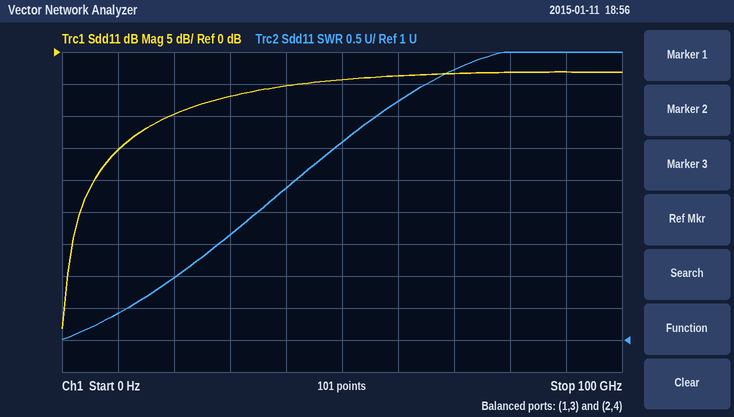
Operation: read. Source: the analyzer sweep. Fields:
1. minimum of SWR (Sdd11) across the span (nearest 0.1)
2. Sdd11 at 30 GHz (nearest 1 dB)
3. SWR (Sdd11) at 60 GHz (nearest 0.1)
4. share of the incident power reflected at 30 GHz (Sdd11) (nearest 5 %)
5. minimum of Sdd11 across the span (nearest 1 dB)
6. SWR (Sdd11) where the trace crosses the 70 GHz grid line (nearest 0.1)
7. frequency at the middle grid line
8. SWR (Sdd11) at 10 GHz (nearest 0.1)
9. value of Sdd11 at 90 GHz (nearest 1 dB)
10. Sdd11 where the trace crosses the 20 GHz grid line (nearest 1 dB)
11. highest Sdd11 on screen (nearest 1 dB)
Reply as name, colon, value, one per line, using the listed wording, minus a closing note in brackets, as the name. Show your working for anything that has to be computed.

minimum of SWR (Sdd11) across the span: 1.0
Sdd11 at 30 GHz: -7 dB
SWR (Sdd11) at 60 GHz: 4.7
share of the incident power reflected at 30 GHz (Sdd11): 10^(-7/10) ≈ 20 %
minimum of Sdd11 across the span: -43 dB
SWR (Sdd11) where the trace crosses the 70 GHz grid line: 5.2
frequency at the middle grid line: 50 GHz
SWR (Sdd11) at 10 GHz: 1.4
value of Sdd11 at 90 GHz: -3 dB
Sdd11 where the trace crosses the 20 GHz grid line: -10 dB
highest Sdd11 on screen: -3 dB
